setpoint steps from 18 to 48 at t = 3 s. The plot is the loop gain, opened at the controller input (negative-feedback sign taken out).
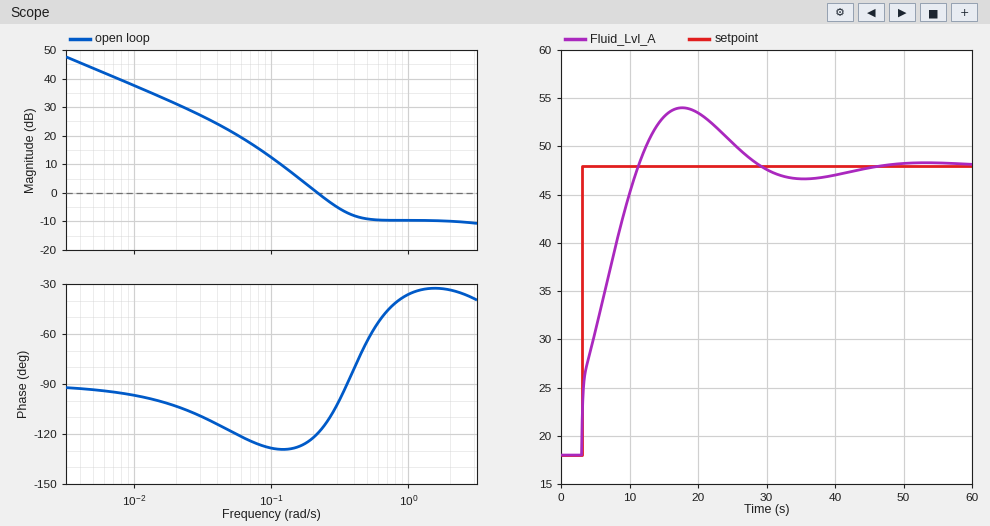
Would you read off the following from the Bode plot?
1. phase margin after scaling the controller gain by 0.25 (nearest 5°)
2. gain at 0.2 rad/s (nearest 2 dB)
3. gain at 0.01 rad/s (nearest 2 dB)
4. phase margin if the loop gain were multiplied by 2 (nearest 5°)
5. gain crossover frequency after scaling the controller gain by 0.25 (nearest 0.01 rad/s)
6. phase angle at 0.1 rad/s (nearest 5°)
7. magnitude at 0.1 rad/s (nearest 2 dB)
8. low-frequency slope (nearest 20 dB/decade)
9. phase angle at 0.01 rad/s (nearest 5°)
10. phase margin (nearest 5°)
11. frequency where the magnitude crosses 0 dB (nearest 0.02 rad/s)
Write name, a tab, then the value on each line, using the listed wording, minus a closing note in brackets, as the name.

phase margin after scaling the controller gain by 0.25	50°
gain at 0.2 rad/s	2 dB
gain at 0.01 rad/s	38 dB
phase margin if the loop gain were multiplied by 2	85°
gain crossover frequency after scaling the controller gain by 0.25	0.10 rad/s
phase angle at 0.1 rad/s	-130°
magnitude at 0.1 rad/s	12 dB
low-frequency slope	-20 dB/decade
phase angle at 0.01 rad/s	-95°
phase margin	60°
frequency where the magnitude crosses 0 dB	0.22 rad/s
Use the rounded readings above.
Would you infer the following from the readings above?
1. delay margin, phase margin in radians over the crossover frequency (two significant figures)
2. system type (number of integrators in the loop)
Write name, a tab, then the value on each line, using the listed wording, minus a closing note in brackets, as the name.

delay margin, phase margin in radians over the crossover frequency	4.8 s
system type	1
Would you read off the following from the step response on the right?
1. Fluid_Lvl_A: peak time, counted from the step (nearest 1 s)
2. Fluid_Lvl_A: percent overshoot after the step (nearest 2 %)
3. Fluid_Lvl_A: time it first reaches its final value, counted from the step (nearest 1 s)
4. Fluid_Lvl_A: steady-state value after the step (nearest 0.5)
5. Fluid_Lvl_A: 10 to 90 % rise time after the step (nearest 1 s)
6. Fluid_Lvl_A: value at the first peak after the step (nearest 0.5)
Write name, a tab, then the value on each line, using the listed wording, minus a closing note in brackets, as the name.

Fluid_Lvl_A: peak time, counted from the step	15 s
Fluid_Lvl_A: percent overshoot after the step	20 %
Fluid_Lvl_A: time it first reaches its final value, counted from the step	8 s
Fluid_Lvl_A: steady-state value after the step	48.0
Fluid_Lvl_A: 10 to 90 % rise time after the step	7 s
Fluid_Lvl_A: value at the first peak after the step	54.0
